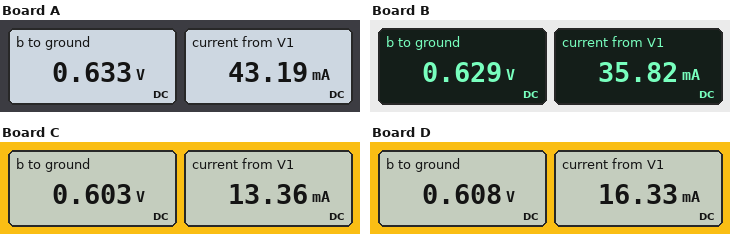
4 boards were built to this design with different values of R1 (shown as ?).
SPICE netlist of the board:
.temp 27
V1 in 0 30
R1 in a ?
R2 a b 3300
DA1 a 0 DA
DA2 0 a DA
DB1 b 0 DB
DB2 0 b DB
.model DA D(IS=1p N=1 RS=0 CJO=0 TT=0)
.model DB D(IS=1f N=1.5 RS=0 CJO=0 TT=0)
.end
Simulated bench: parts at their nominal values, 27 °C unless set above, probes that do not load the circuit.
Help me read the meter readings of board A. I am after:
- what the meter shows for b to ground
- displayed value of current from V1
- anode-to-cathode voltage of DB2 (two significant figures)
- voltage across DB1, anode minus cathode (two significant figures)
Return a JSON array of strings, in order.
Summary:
["0.633 V", "43.19 mA", "-630 mV", "630 mV"]
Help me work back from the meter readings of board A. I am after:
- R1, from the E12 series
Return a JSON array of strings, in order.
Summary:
["680 Ω"]
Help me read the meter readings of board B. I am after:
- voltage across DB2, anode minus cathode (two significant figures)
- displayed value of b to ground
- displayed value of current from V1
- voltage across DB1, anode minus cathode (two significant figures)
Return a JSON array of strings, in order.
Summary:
["-630 mV", "0.629 V", "35.82 mA", "630 mV"]
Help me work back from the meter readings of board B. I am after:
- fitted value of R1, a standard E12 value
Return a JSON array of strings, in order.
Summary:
["820 Ω"]
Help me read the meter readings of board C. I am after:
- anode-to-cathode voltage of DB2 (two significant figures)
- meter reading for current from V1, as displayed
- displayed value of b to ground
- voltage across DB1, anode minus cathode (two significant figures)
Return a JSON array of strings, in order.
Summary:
["-600 mV", "13.36 mA", "0.603 V", "600 mV"]
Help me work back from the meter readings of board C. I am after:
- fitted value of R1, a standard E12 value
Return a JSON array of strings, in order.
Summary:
["2.2 kΩ"]
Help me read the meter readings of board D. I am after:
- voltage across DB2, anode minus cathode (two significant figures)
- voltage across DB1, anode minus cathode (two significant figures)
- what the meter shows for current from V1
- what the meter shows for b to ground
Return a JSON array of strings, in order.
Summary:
["-610 mV", "610 mV", "16.33 mA", "0.608 V"]
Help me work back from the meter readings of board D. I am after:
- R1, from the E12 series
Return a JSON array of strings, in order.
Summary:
["1.8 kΩ"]
